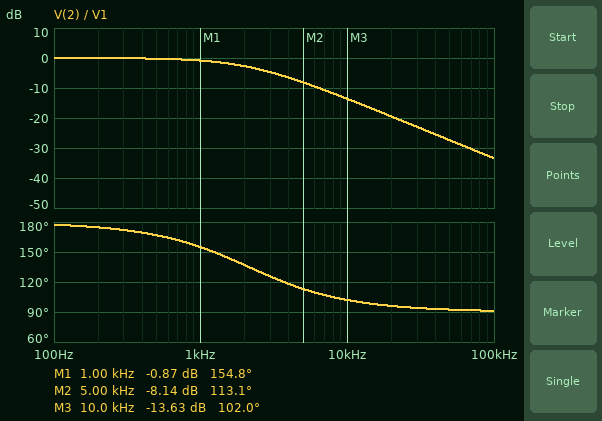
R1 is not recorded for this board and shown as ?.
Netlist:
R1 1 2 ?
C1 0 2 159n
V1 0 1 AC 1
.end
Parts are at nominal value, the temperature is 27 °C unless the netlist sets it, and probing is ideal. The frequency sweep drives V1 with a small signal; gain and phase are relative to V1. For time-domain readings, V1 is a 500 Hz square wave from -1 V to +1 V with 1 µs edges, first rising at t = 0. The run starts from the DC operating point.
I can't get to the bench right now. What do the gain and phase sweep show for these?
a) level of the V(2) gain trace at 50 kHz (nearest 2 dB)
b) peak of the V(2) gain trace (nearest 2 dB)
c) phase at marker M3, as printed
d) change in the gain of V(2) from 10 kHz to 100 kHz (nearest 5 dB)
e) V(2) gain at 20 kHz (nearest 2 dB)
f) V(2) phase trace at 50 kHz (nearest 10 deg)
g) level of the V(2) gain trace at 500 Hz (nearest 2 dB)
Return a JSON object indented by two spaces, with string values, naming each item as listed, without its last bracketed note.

{
  "level of the V(2) gain trace at 50 kHz": "-28 dB",
  "peak of the V(2) gain trace": "0 dB",
  "phase at marker M3, as printed": "102.0 deg",
  "change in the gain of V(2) from 10 kHz to 100 kHz": "-20 dB",
  "V(2) gain at 20 kHz": "-20 dB",
  "V(2) phase trace at 50 kHz": "90 deg",
  "level of the V(2) gain trace at 500 Hz": "0 dB"
}
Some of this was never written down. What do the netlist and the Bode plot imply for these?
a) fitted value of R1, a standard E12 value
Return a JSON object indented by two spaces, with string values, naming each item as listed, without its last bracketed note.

{
  "fitted value of R1, a standard E12 value": "470 Ω"
}
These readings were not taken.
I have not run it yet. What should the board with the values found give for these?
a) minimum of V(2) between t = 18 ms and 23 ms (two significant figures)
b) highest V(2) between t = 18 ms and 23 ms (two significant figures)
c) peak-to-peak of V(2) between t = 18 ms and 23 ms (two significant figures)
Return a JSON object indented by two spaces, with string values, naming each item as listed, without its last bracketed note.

{
  "minimum of V(2) between t = 18 ms and 23 ms": "-1.0 V",
  "highest V(2) between t = 18 ms and 23 ms": "1.0 V",
  "peak-to-peak of V(2) between t = 18 ms and 23 ms": "2.0 V"
}
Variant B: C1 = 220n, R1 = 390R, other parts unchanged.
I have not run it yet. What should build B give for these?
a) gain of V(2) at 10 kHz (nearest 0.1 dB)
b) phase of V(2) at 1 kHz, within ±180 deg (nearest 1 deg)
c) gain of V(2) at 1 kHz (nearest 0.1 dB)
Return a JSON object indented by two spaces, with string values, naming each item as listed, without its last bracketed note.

{
  "gain of V(2) at 10 kHz": "-14.8 dB",
  "phase of V(2) at 1 kHz, within ±180 deg": "152 deg",
  "gain of V(2) at 1 kHz": "-1.1 dB"
}
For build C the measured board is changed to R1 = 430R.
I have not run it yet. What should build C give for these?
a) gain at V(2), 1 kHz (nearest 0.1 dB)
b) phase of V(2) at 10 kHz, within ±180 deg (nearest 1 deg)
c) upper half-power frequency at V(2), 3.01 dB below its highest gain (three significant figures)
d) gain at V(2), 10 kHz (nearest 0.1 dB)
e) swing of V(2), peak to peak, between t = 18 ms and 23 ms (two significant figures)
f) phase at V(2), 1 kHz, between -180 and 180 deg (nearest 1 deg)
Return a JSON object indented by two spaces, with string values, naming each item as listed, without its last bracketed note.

{
  "gain at V(2), 1 kHz": "-0.7 dB",
  "phase of V(2) at 10 kHz, within ±180 deg": "103 deg",
  "upper half-power frequency at V(2), 3.01 dB below its highest gain": "2.33 kHz",
  "gain at V(2), 10 kHz": "-12.9 dB",
  "swing of V(2), peak to peak, between t = 18 ms and 23 ms": "2.0 V",
  "phase at V(2), 1 kHz, between -180 and 180 deg": "157 deg"
}
